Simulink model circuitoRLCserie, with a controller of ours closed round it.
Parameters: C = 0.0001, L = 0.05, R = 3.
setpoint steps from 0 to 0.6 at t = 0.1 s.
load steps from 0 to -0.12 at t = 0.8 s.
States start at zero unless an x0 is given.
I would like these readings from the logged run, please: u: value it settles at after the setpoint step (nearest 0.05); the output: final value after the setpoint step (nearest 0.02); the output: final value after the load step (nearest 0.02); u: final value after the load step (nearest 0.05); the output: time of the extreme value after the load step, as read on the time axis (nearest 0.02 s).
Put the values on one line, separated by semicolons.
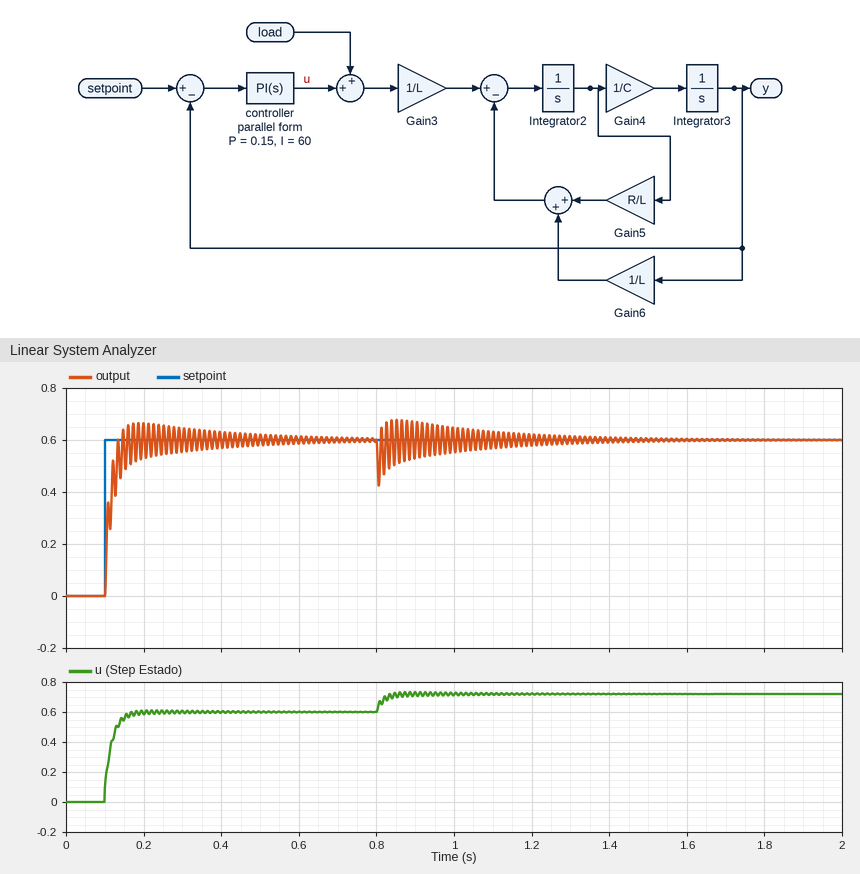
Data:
0.60; 0.60; 0.60; 0.70; 0.80 s
